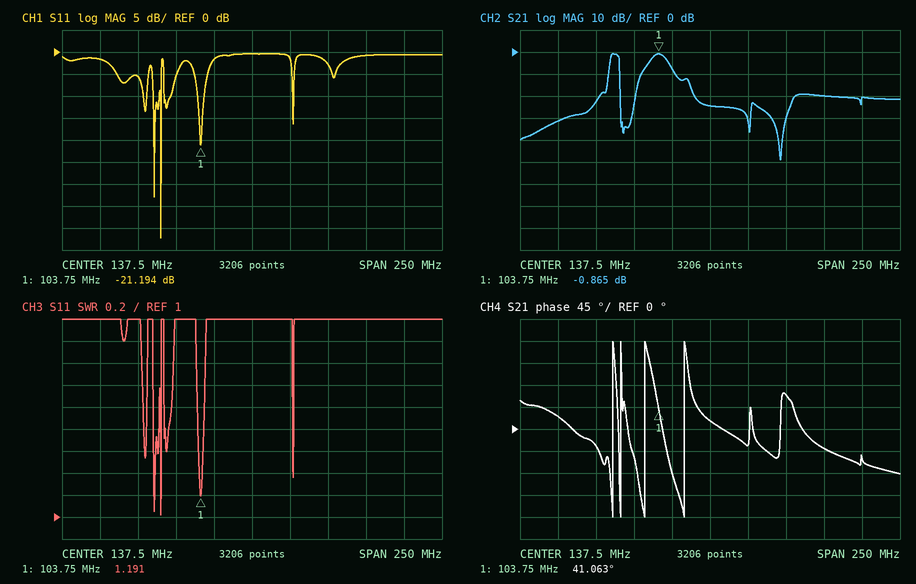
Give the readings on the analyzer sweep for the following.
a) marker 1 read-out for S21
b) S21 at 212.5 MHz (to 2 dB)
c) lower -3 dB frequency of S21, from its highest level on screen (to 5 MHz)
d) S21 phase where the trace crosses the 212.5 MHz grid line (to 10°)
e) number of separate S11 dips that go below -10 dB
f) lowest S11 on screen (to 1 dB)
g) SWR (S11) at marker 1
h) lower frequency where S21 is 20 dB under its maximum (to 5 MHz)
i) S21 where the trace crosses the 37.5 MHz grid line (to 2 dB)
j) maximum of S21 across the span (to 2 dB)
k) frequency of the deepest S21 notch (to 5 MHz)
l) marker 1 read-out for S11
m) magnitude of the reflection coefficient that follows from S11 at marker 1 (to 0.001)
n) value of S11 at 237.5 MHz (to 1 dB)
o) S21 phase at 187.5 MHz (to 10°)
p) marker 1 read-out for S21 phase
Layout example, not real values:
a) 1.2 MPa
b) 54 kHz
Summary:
a) -0.865 dB
b) -20 dB
c) 70 MHz
d) -40°
e) 6
f) -42 dB
g) 1.191
h) 65 MHz
i) -32 dB
j) 0 dB
k) 185 MHz
l) -21.194 dB
m) 0.087
n) -1 dB
o) 70°
p) 41.063°
